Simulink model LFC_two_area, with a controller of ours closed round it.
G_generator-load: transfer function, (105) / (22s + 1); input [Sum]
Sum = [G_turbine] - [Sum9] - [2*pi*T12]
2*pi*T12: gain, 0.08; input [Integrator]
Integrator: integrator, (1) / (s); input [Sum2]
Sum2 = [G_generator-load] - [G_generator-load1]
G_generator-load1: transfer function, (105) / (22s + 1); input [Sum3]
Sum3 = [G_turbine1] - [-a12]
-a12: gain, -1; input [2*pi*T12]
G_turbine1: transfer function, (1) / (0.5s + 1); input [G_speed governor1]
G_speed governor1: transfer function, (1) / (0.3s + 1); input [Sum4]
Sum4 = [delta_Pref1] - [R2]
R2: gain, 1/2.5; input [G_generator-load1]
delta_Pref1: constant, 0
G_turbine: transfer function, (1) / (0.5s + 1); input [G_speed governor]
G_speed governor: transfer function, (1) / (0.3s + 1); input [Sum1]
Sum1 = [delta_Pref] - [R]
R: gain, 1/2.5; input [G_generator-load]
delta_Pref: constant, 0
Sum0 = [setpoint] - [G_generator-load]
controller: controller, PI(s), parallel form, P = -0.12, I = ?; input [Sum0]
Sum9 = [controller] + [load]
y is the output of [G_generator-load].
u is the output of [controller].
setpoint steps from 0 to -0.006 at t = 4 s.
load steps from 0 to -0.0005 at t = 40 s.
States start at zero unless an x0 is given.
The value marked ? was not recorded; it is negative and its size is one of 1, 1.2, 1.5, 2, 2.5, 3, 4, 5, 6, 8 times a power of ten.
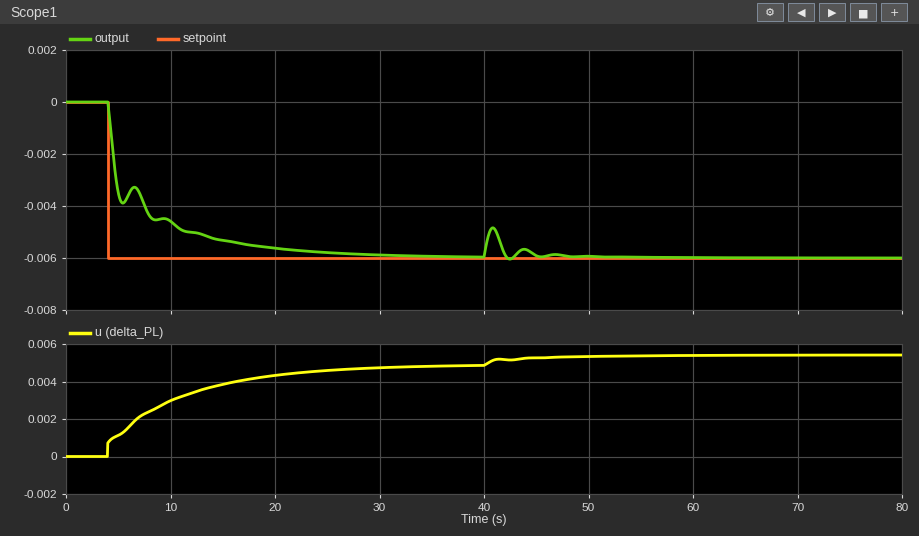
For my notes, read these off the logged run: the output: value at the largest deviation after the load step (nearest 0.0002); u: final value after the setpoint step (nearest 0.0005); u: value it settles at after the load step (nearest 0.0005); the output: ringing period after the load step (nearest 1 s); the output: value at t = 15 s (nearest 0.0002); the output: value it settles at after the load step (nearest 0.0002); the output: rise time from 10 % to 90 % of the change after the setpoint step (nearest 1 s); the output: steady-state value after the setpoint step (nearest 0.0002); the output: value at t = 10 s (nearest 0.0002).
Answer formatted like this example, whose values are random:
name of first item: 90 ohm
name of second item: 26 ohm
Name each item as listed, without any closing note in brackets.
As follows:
the output: value at the largest deviation after the load step: -0.0048
u: final value after the setpoint step: 0.0050
u: value it settles at after the load step: 0.0055
the output: ringing period after the load step: 3 s
the output: value at t = 15 s: -0.0054
the output: value it settles at after the load step: -0.0060
the output: rise time from 10 % to 90 % of the change after the setpoint step: 12 s
the output: steady-state value after the setpoint step: -0.0060
the output: value at t = 10 s: -0.0046
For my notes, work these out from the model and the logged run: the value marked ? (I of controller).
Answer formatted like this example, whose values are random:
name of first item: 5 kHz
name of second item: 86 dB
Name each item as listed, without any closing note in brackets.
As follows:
the value marked ?: -0.2
